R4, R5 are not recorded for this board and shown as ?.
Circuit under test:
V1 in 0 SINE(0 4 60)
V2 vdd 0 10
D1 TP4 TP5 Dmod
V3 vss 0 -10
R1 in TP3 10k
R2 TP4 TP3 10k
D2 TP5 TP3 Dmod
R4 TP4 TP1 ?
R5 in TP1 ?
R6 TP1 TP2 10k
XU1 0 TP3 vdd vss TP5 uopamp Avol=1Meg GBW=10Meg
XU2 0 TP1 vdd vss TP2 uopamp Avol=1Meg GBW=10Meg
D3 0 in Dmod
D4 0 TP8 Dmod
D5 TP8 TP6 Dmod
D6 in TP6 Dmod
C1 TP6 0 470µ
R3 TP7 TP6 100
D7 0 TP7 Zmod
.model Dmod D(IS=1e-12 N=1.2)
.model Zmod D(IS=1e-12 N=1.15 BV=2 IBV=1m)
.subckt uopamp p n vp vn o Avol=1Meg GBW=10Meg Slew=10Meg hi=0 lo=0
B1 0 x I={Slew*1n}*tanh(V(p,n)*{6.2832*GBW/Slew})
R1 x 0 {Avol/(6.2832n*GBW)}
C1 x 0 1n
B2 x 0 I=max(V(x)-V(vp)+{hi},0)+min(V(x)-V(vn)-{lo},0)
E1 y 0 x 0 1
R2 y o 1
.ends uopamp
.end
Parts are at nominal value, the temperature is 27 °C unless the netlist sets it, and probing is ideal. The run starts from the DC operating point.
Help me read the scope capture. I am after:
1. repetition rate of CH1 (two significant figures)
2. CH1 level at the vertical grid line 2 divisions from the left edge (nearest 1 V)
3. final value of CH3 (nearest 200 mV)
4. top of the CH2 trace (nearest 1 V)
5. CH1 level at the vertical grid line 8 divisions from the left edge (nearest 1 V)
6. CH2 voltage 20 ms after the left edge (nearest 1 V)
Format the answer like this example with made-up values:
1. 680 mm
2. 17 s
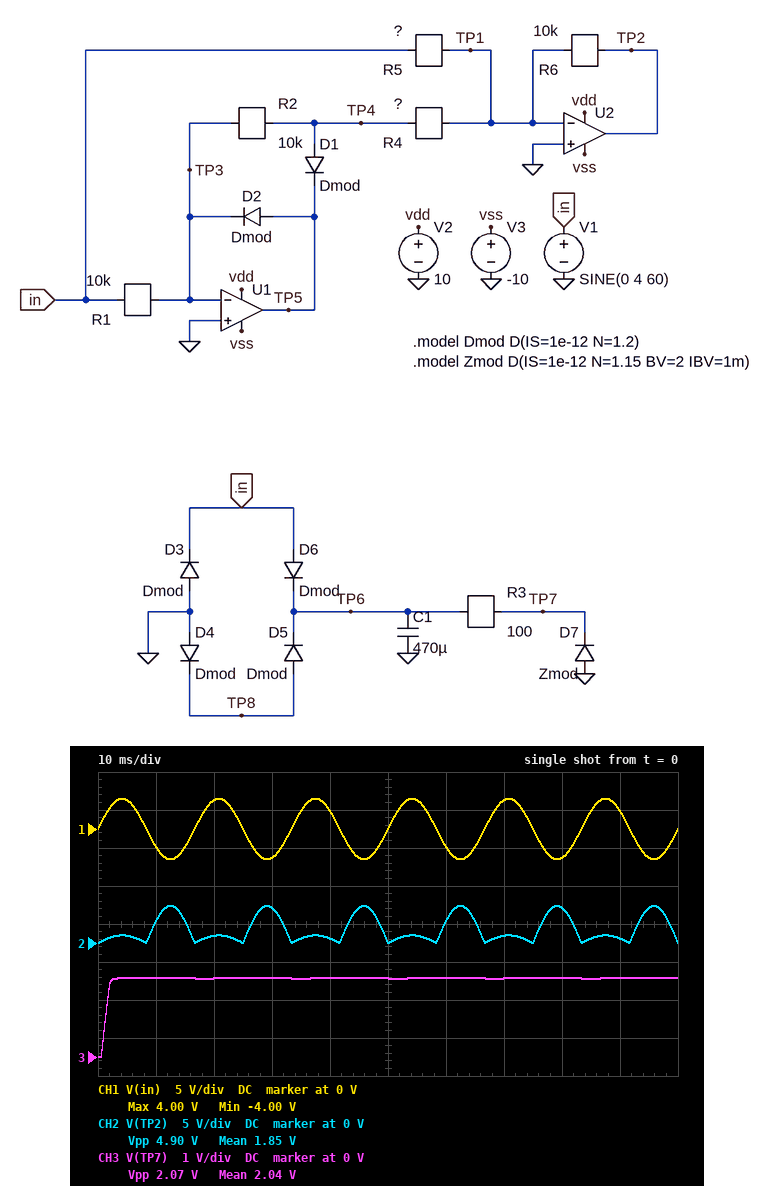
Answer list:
1. 60 Hz
2. 4 V
3. 2.0 V
4. 5 V
5. -4 V
6. 1 V
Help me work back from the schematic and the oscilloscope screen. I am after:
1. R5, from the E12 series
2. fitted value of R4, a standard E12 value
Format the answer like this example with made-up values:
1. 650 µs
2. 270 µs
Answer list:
1. 8.2 kΩ
2. 6.8 kΩ
